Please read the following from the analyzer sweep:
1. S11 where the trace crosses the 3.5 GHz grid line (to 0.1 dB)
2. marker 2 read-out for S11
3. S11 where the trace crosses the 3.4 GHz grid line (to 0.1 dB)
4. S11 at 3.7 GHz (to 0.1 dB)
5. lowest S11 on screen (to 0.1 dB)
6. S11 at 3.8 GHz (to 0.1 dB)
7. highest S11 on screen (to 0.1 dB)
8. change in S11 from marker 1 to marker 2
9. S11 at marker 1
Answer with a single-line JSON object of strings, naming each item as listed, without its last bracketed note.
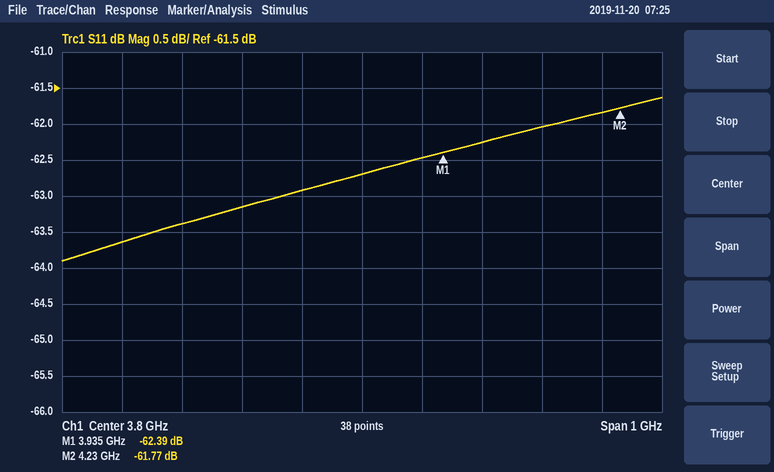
{"S11 where the trace crosses the 3.5 GHz grid line": "-63.4 dB", "marker 2 read-out for S11": "-61.77 dB", "S11 where the trace crosses the 3.4 GHz grid line": "-63.6 dB", "S11 at 3.7 GHz": "-62.9 dB", "lowest S11 on screen": "-63.9 dB", "S11 at 3.8 GHz": "-62.7 dB", "highest S11 on screen": "-61.6 dB", "change in S11 from marker 1 to marker 2": "0.62 dB", "S11 at marker 1": "-62.39 dB"}
